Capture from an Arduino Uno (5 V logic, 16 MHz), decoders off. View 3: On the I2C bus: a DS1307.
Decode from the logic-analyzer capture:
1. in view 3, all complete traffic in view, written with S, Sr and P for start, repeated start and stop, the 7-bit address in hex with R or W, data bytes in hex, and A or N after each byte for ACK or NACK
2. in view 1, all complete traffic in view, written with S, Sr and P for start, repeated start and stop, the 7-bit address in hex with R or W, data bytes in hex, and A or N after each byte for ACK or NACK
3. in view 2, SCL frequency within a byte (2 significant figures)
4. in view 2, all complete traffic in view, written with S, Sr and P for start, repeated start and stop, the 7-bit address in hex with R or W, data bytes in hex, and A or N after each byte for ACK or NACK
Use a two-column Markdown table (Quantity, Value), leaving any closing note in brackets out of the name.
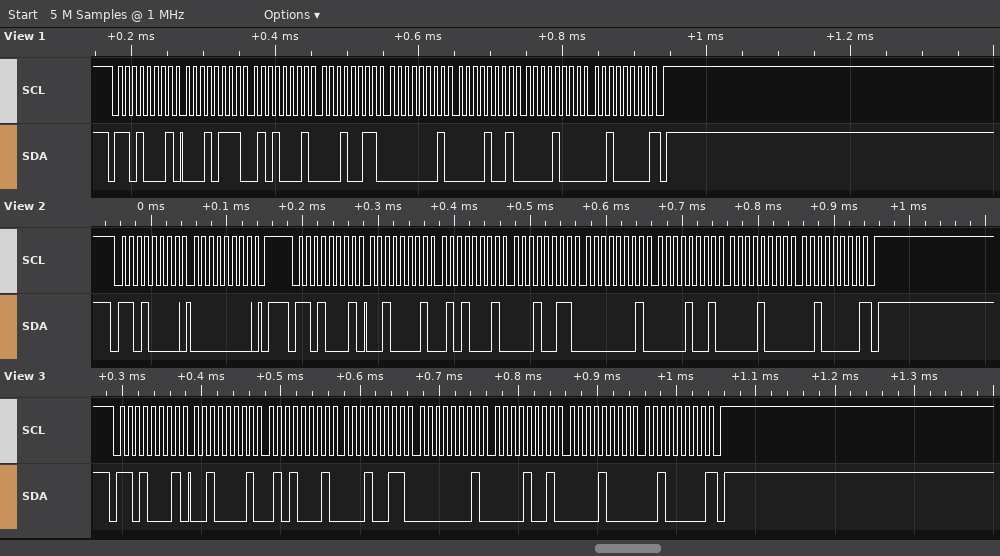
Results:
| Quantity | Value |
|---|---|
| in view 3, all complete traffic in view, written with S, Sr and P for start, repeated start and stop, the 7-bit address in hex with R or W, data bytes in hex, and A or N after each byte for ACK or NACK | S 68R A 21 A 51 A 13 A 01 A 09 A 08 A 20 N P |
| in view 1, all complete traffic in view, written with S, Sr and P for start, repeated start and stop, the 7-bit address in hex with R or W, data bytes in hex, and A or N after each byte for ACK or NACK | S 68R A 17 A 51 A 13 A 01 A 09 A 08 A 20 N P |
| in view 2, SCL frequency within a byte | 100 kHz |
| in view 2, all complete traffic in view, written with S, Sr and P for start, repeated start and stop, the 7-bit address in hex with R or W, data bytes in hex, and A or N after each byte for ACK or NACK | S 68W A 00 A P S 68R A 21 A 51 A 13 A 01 A 09 A 08 A 20 N P |
